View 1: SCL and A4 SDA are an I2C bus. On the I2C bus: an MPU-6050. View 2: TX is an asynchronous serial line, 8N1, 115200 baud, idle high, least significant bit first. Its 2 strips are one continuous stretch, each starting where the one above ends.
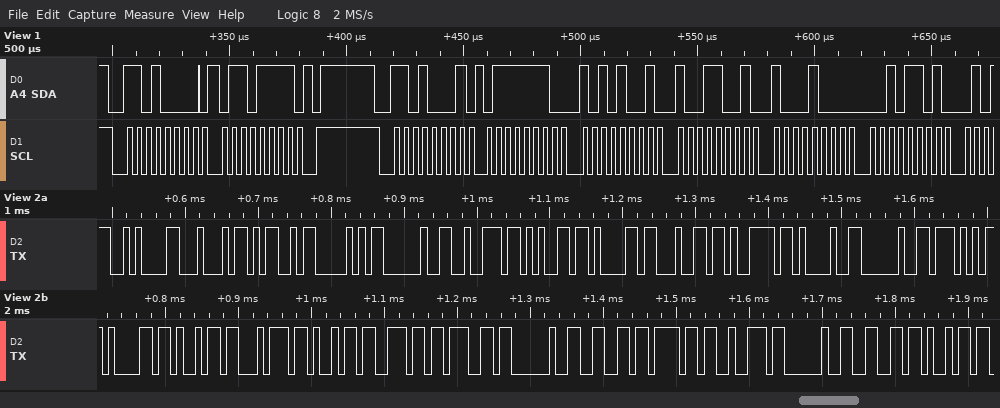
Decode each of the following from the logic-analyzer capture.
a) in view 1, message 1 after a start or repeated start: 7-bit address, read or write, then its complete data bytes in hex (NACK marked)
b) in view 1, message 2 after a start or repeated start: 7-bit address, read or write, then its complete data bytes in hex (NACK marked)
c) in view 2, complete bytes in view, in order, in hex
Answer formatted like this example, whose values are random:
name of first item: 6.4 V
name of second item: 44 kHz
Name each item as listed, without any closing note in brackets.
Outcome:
in view 1, message 1 after a start or repeated start: 7-bit address, read or write, then its complete data bytes in hex: 0x68 write: 6F
in view 1, message 2 after a start or repeated start: 7-bit address, read or write, then its complete data bytes in hex: 0x68 read: 7E A9 99 88 2D
in view 2, complete bytes in view, in order, in hex: 0A 44 4D 50 20 72 65 61 64 79 21 20 57 61 69 74 69 6E 67 20 66 6F 72 20 66 69
